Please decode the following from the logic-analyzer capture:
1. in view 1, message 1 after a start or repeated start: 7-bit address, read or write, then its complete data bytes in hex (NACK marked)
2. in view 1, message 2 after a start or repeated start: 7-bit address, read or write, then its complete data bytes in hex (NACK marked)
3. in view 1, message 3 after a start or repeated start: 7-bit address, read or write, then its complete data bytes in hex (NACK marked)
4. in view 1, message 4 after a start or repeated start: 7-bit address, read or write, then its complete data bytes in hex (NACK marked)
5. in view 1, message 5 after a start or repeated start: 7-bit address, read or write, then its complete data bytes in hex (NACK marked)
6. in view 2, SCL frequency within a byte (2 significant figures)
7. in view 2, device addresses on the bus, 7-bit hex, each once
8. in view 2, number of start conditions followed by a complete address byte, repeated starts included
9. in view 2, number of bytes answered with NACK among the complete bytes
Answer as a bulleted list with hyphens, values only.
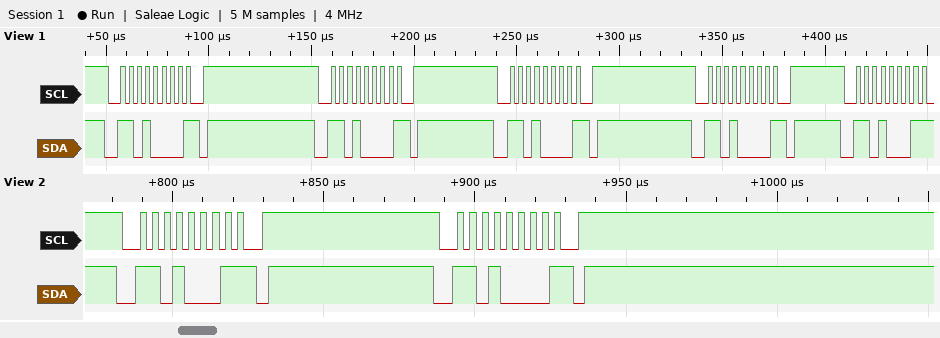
- 0x68 write NACK
- 0x68 write NACK
- 0x68 write NACK
- 0x68 write NACK
- 0x68 read NACK
- 250 kHz
- 0x68
- 2
- 2
